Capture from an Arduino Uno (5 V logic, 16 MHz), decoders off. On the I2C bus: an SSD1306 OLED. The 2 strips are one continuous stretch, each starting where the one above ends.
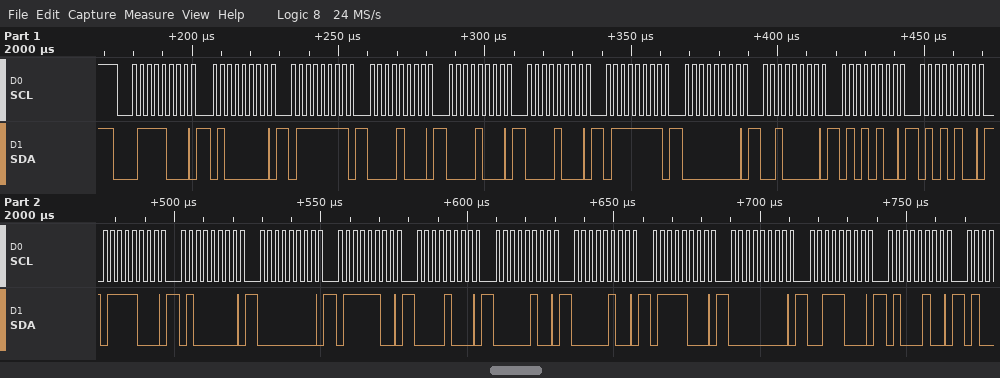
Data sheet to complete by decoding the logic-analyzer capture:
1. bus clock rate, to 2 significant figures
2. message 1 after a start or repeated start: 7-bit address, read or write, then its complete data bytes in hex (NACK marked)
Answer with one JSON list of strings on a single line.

["400 kHz", "0x3C write: 40 7F 08 08 08 7F 00 20 54 54 78 40 00 7C 08 04 04 78 00 38 44"]
